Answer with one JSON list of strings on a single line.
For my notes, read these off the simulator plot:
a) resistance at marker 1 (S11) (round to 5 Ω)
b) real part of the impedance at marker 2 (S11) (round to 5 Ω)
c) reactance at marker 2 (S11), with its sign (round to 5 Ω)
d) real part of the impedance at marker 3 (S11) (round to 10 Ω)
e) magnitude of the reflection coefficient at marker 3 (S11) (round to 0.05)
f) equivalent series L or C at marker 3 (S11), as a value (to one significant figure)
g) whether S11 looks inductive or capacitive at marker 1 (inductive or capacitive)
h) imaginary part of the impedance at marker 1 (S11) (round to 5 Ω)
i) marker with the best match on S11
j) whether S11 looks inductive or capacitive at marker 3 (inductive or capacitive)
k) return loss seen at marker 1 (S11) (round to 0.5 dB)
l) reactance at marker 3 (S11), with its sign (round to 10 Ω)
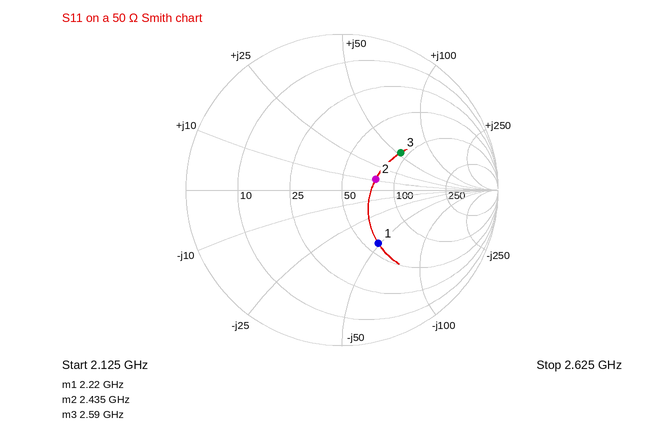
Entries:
["60 Ω", "75 Ω", "+10 Ω", "90 Ω", "0.45", "3 nH", "capacitive", "-50 Ω", "marker 2", "inductive", "7.5 dB", "+50 Ω"]
